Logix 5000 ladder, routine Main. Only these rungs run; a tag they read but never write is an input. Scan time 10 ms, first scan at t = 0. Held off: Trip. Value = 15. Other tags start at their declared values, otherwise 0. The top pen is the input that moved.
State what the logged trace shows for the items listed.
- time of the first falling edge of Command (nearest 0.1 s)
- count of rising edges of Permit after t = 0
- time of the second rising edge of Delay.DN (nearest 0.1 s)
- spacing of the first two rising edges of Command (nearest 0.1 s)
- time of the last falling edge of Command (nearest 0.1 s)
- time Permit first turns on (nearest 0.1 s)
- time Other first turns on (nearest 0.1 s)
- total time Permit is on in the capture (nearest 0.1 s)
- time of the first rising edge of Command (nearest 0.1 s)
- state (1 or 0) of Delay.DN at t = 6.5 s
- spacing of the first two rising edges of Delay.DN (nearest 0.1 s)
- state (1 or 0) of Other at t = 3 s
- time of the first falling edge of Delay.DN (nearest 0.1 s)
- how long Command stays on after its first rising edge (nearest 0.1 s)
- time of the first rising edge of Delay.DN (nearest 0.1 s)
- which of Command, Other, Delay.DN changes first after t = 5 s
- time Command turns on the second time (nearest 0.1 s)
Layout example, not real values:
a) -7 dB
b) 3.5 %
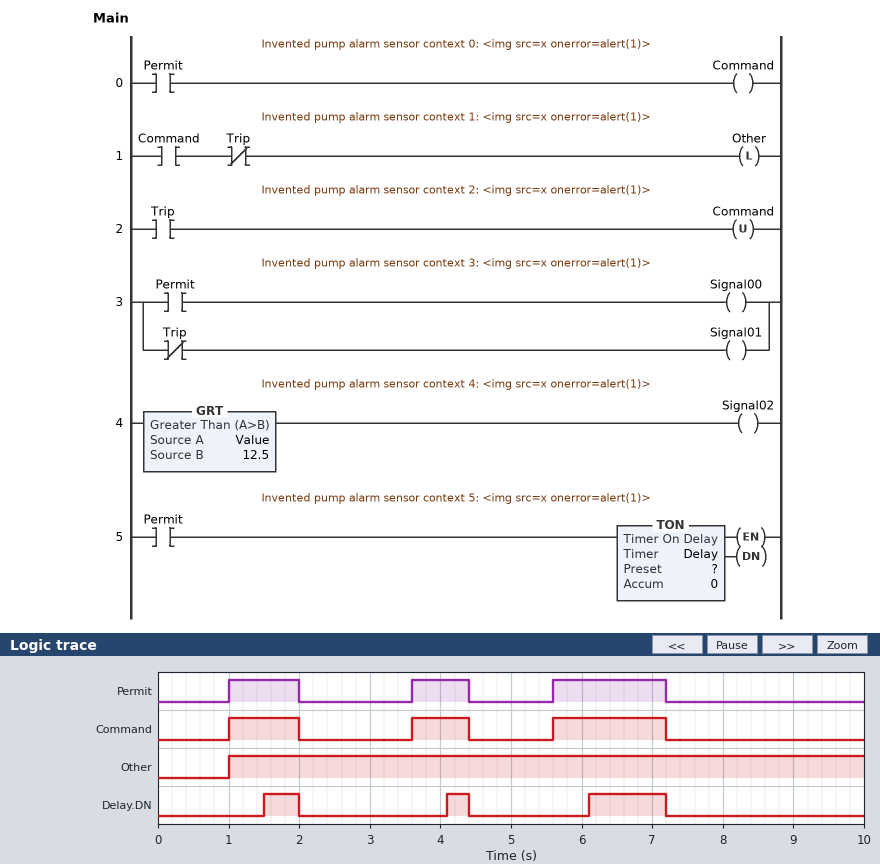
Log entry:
a) 2.0 s
b) 3
c) 4.1 s
d) 2.6 s
e) 7.2 s
f) 1.0 s
g) 1.0 s
h) 3.4 s
i) 1.0 s
j) 1
k) 2.6 s
l) 1
m) 2.0 s
n) 1.0 s
o) 1.5 s
p) Command
q) 3.6 s
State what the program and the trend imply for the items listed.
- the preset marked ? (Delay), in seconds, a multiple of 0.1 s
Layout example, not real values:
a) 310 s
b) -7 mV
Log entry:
a) 0.5 s
